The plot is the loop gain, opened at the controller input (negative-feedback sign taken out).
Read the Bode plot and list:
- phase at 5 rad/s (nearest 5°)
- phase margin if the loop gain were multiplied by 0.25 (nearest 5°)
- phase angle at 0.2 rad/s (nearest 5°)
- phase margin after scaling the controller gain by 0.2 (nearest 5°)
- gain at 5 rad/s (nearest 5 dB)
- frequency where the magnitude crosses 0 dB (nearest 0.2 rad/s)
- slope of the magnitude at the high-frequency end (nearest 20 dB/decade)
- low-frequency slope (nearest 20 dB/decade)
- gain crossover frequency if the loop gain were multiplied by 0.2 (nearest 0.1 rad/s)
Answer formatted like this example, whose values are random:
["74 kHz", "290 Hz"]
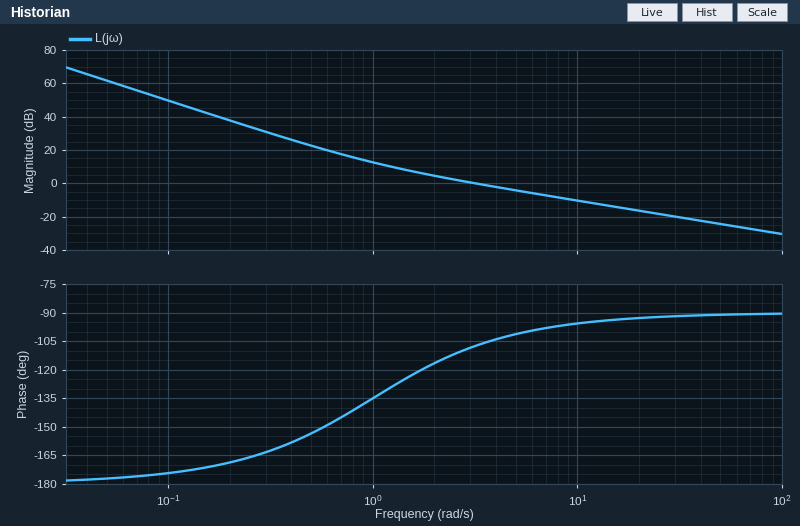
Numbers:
["-100°", "45°", "-170°", "40°", "-5 dB", "3.2 rad/s", "-20 dB/decade", "-40 dB/decade", "0.9 rad/s"]
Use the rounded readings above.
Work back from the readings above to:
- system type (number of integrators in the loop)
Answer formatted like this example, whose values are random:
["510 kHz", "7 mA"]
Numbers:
["2"]
